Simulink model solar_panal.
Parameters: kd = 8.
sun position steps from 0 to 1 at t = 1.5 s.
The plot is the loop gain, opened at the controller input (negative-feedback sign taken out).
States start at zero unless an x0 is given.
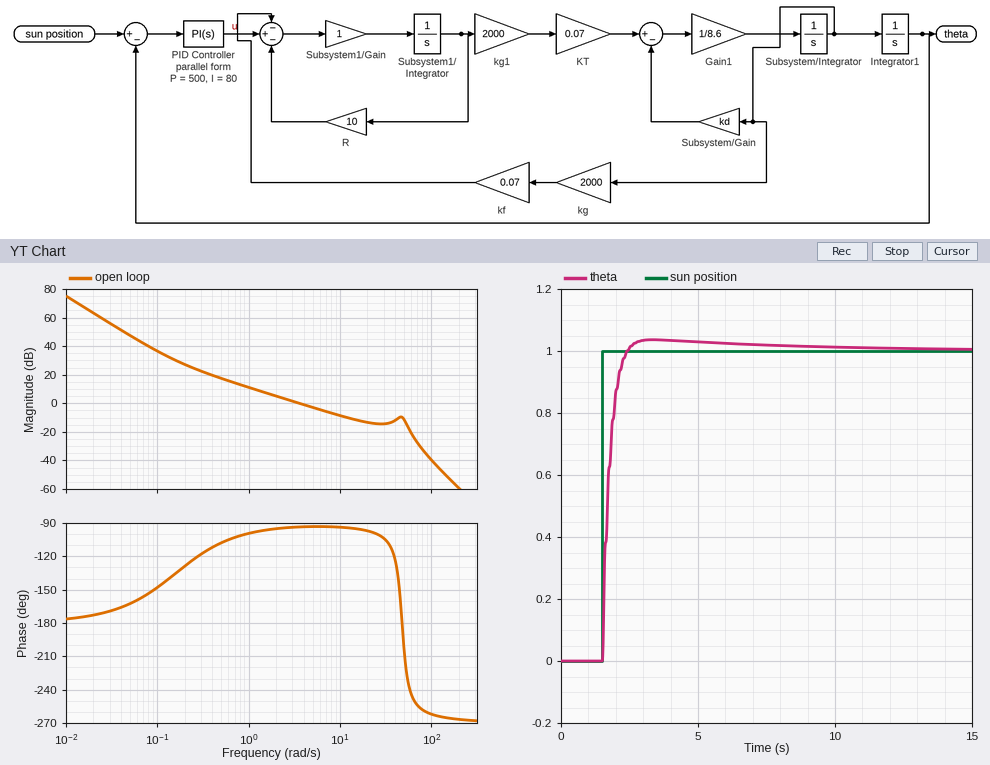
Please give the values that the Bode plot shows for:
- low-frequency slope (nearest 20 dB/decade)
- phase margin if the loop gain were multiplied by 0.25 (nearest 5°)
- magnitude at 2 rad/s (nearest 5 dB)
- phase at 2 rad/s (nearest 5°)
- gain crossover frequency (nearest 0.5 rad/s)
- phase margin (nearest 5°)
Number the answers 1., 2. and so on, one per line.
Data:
1. -40 dB/decade
2. 80°
3. 5 dB
4. -95°
5. 3.5 rad/s
6. 85°
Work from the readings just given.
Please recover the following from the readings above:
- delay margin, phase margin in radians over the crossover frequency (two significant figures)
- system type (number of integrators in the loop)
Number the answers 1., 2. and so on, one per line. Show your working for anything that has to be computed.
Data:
1. 85 × π / 180 / 3.5 = 0.42 s
2. 2
